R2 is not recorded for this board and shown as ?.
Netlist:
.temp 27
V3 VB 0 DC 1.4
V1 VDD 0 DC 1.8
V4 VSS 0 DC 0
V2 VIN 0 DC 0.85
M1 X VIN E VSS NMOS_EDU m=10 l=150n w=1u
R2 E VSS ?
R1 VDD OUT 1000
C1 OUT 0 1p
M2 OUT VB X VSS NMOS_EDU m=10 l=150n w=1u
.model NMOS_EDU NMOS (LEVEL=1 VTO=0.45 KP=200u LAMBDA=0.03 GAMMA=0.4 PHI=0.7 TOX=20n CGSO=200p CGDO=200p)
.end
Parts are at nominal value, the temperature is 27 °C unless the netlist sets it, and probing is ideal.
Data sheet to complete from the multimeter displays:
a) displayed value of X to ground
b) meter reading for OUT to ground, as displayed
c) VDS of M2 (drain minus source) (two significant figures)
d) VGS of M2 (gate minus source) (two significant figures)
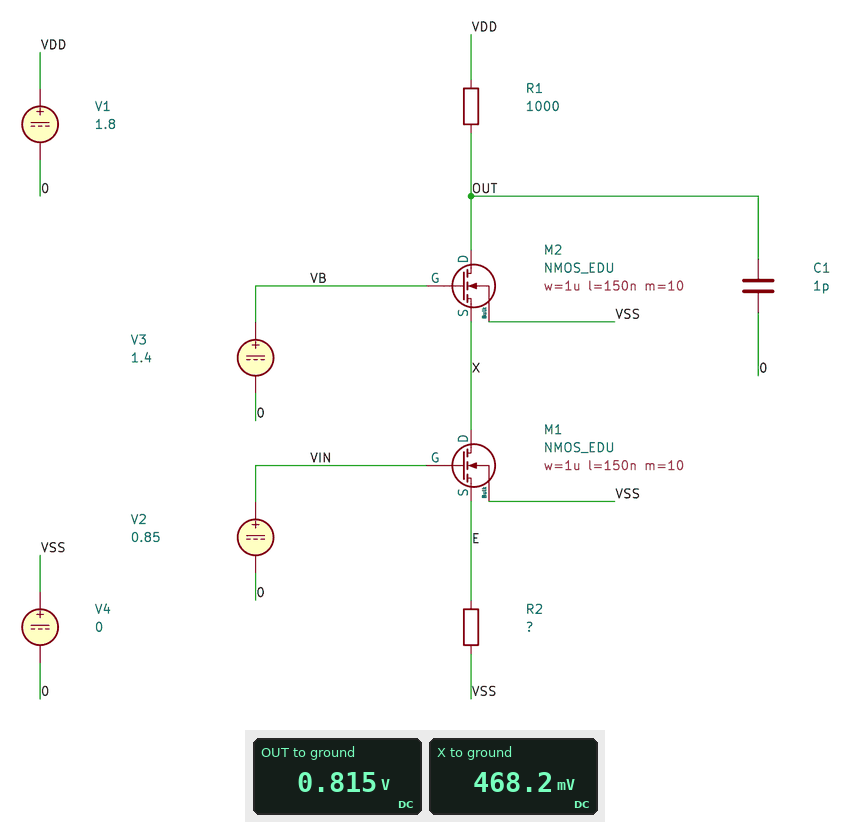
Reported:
468.2 mV
0.815 V
350 mV
930 mV
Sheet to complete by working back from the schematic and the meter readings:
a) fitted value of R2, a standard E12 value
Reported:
15 Ω
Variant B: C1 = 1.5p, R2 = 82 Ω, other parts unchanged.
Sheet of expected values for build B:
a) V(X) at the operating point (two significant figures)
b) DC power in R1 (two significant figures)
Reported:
520 mV
520 µW
